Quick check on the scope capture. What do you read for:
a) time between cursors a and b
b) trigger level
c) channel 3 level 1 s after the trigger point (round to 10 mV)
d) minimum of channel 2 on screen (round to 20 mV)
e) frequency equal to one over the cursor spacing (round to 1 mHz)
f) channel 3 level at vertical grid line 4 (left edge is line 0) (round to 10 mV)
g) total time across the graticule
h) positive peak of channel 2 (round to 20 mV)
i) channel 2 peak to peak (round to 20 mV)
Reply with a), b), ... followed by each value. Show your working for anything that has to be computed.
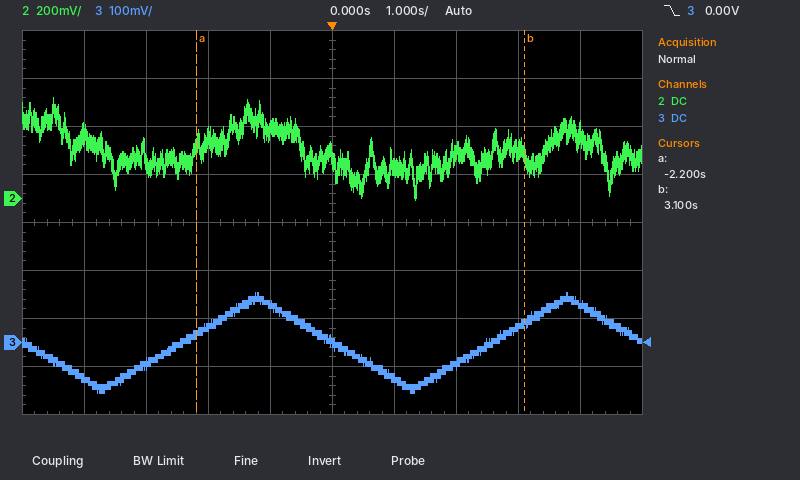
a) 3.1 s − (-2.2 s) = 5.3 s
b) 0.00 V
c) -70 mV
d) 0 mV
e) 1 / 5.3 s ≈ 189 mHz
f) 80 mV
g) 10 s
h) 420 mV
i) 420 mV − (0 mV) = 420 mV
